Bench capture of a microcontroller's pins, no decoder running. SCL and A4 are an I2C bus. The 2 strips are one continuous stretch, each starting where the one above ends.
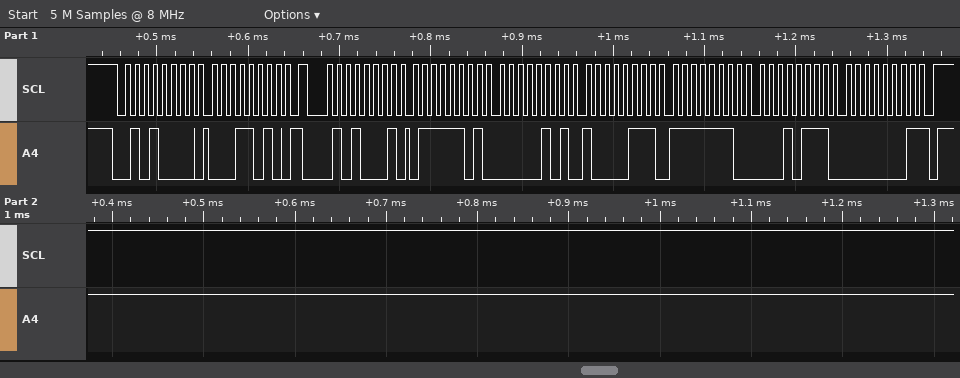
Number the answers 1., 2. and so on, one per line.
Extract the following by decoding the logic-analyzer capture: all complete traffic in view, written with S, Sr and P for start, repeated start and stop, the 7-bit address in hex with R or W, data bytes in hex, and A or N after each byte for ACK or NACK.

1. S 28W A 1A A Sr 28R A 7D A 05 A 87 A FE A 17 A 01 N P
